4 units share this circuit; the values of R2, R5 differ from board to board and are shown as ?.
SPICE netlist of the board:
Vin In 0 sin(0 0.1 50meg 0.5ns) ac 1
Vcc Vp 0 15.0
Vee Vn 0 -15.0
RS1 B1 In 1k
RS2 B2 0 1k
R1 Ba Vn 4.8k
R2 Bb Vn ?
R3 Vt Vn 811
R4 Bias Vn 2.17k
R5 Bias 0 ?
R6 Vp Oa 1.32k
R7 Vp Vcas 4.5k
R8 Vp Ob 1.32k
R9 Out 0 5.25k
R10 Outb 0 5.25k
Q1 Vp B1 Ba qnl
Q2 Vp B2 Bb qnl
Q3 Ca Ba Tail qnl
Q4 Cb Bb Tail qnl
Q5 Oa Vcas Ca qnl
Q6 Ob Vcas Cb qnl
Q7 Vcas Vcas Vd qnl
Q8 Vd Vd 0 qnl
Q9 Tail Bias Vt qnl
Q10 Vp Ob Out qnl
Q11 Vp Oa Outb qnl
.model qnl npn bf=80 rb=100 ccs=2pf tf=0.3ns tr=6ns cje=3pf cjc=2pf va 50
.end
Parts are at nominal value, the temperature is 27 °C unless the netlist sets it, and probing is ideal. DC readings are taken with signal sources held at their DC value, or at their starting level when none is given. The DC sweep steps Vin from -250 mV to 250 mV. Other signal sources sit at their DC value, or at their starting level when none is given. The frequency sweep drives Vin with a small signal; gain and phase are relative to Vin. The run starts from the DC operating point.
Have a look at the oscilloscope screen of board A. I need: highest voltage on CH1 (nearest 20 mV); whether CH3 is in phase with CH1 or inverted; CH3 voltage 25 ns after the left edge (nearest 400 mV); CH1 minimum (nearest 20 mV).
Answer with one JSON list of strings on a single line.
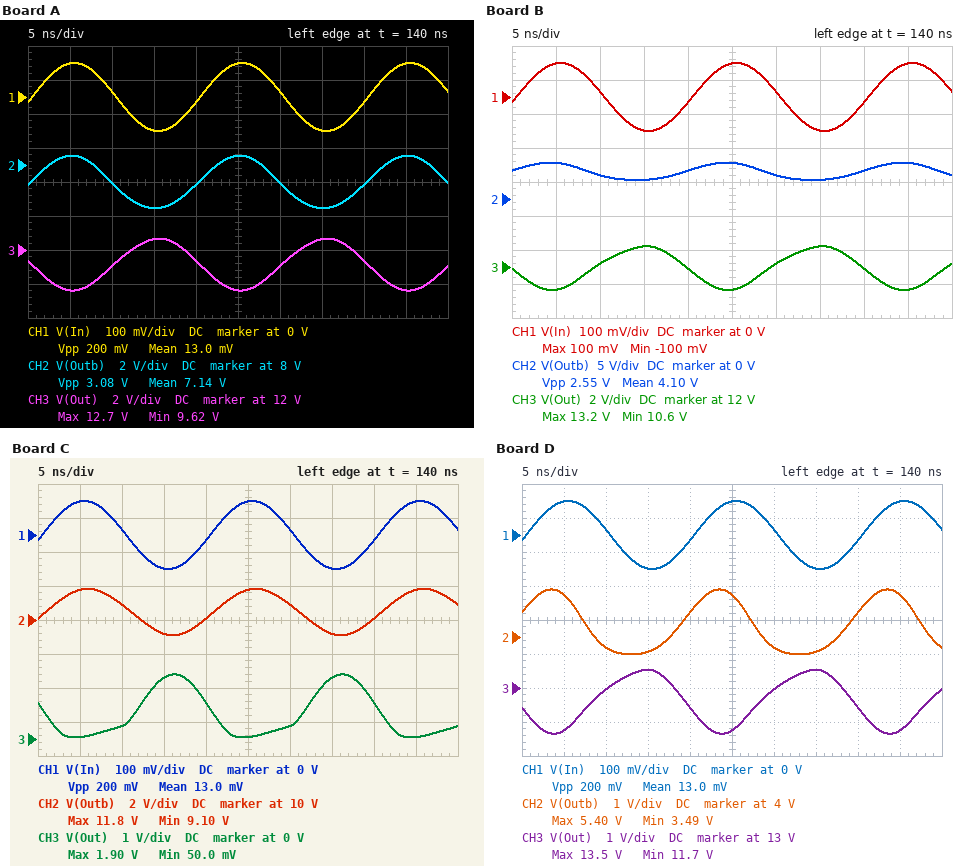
["100 mV", "inverted", "9.6 V", "-100 mV"]
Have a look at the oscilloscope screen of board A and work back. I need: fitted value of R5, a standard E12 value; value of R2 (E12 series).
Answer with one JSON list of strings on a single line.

["2.2 kΩ", "2.7 kΩ"]
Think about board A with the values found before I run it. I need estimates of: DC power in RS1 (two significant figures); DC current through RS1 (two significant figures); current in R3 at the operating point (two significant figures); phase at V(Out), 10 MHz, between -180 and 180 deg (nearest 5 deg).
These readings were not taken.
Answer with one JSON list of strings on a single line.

["830 nW", "29 µA", "8.0 mA", "-40 deg"]
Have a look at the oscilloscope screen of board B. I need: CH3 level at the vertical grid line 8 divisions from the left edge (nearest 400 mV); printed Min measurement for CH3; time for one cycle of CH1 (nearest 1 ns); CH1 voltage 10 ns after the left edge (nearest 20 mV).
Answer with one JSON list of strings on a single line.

["12.0 V", "10.6 V", "20 ns", "20 mV"]
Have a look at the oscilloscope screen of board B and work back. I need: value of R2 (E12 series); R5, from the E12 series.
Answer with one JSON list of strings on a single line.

["1.8 kΩ", "1.5 kΩ"]
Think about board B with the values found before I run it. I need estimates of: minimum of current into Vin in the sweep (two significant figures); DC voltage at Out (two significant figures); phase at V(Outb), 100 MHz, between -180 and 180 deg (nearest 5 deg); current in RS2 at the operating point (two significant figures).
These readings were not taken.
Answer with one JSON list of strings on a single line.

["-30 µA", "13 V", "-40 deg", "75 µA"]
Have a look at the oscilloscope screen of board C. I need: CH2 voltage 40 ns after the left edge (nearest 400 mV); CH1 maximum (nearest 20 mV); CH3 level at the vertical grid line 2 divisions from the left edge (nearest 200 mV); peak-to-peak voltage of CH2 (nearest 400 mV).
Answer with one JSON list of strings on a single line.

["10.0 V", "100 mV", "400 mV", "2.8 V"]
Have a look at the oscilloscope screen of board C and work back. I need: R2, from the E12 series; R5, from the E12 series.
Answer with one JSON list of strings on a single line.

["15 kΩ", "560 Ω"]
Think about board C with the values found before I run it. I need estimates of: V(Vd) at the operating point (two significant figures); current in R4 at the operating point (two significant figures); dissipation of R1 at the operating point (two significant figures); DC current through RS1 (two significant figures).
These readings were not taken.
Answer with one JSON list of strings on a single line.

["800 mV", "5.5 mA", "42 mW", "28 µA"]
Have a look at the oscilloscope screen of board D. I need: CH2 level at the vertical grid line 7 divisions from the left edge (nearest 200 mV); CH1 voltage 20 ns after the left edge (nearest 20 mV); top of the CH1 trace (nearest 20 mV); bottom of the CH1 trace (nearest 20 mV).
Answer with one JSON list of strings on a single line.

["3.6 V", "-20 mV", "100 mV", "-100 mV"]
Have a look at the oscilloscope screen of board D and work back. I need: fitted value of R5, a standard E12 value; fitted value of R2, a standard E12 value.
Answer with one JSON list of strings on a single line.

["1.8 kΩ", "1.5 kΩ"]
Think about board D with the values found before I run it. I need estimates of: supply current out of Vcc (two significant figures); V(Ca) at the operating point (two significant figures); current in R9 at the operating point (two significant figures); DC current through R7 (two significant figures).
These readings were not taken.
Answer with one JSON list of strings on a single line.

["27 mA", "770 mV", "2.6 mA", "3.0 mA"]
